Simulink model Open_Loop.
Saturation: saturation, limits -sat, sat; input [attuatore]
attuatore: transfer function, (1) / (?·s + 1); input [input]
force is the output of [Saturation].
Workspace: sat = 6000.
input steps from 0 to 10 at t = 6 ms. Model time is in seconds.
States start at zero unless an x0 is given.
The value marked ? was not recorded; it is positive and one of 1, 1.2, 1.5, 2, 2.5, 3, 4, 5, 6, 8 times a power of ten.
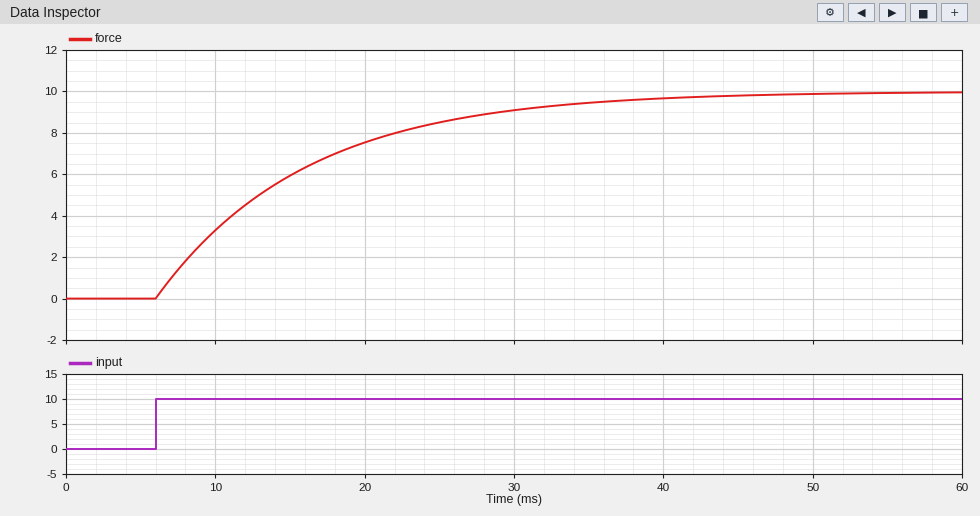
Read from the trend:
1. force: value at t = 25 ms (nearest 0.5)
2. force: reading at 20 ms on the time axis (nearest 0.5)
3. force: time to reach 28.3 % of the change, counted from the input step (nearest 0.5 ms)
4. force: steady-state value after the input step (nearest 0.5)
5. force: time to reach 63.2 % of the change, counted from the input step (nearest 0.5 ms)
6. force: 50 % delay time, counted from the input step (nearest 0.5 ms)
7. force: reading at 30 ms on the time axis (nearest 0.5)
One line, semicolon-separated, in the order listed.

8.5; 7.5; 3.5 ms; 10.0; 10.0 ms; 7.0 ms; 9.0
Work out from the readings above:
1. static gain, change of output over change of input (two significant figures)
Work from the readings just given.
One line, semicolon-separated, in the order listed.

1.0
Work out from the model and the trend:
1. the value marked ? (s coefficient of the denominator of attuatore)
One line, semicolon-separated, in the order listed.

0.01
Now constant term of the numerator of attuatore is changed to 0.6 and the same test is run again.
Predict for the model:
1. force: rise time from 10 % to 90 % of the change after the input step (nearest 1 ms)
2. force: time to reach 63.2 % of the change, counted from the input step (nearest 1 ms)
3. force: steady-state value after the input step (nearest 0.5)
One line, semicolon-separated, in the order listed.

22 ms; 10 ms; 6.0
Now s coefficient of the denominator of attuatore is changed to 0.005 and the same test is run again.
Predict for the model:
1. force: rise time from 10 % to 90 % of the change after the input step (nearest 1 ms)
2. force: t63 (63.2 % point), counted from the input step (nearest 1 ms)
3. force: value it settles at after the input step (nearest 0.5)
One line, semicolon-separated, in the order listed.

11 ms; 5 ms; 10.0
